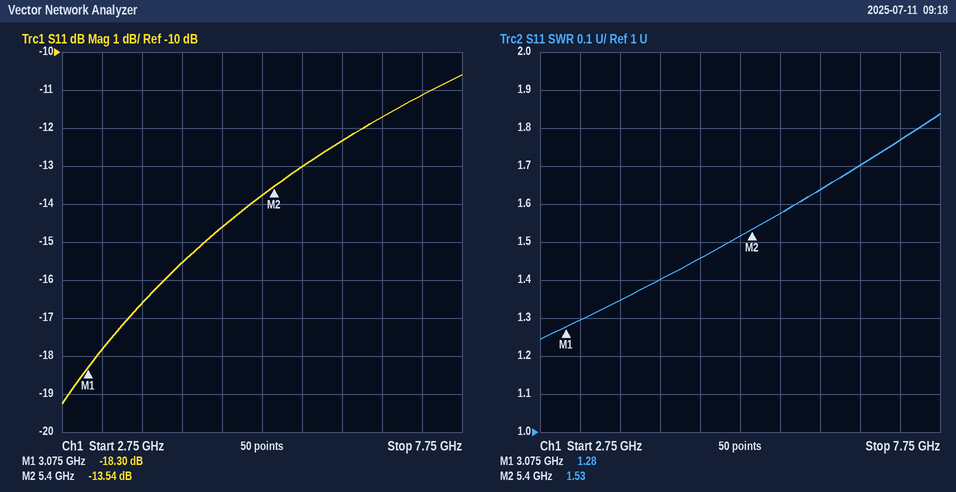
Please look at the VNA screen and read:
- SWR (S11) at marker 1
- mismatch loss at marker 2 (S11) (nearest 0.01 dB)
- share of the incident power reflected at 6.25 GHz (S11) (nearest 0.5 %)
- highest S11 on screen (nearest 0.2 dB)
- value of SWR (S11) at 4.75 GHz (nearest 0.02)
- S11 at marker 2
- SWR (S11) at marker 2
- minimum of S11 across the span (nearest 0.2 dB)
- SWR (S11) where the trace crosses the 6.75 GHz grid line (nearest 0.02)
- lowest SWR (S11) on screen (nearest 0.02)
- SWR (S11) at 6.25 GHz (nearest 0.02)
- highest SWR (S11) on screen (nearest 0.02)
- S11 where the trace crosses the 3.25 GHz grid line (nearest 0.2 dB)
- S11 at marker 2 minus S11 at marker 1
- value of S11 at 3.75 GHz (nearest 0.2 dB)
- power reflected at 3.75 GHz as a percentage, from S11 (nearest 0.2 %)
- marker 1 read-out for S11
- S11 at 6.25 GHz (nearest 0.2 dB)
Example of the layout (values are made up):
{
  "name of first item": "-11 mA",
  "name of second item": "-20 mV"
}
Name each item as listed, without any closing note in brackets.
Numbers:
{
  "SWR (S11) at marker 1": "1.28",
  "mismatch loss at marker 2 (S11)": "0.20 dB",
  "share of the incident power reflected at 6.25 GHz (S11)": "6.0 %",
  "highest S11 on screen": "-10.6 dB",
  "value of SWR (S11) at 4.75 GHz": "1.46",
  "S11 at marker 2": "-13.54 dB",
  "SWR (S11) at marker 2": "1.53",
  "minimum of S11 across the span": "-19.2 dB",
  "SWR (S11) where the trace crosses the 6.75 GHz grid line": "1.70",
  "lowest SWR (S11) on screen": "1.24",
  "SWR (S11) at 6.25 GHz": "1.64",
  "highest SWR (S11) on screen": "1.84",
  "S11 where the trace crosses the 3.25 GHz grid line": "-17.8 dB",
  "S11 at marker 2 minus S11 at marker 1": "4.76 dB",
  "value of S11 at 3.75 GHz": "-16.6 dB",
  "power reflected at 3.75 GHz as a percentage, from S11": "2.2 %",
  "marker 1 read-out for S11": "-18.30 dB",
  "S11 at 6.25 GHz": "-12.4 dB"
}
